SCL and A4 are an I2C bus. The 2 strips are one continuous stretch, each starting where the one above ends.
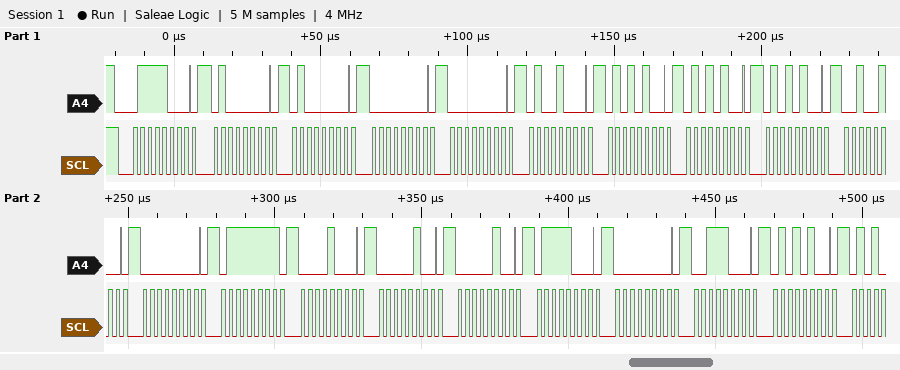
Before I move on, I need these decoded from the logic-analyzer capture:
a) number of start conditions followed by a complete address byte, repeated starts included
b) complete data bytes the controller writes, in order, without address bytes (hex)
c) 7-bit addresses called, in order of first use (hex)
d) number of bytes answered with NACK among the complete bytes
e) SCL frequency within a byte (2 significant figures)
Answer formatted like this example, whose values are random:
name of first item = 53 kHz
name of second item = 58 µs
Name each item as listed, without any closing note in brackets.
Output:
number of start conditions followed by a complete address byte, repeated starts included = 1
complete data bytes the controller writes, in order, without address bytes = 40 40 00 00 48 54 54 54 24 00 7F 08 04 04 78 00 38 54
7-bit addresses called, in order of first use = 0x3C
number of bytes answered with NACK among the complete bytes = 0
SCL frequency within a byte = 400 kHz
